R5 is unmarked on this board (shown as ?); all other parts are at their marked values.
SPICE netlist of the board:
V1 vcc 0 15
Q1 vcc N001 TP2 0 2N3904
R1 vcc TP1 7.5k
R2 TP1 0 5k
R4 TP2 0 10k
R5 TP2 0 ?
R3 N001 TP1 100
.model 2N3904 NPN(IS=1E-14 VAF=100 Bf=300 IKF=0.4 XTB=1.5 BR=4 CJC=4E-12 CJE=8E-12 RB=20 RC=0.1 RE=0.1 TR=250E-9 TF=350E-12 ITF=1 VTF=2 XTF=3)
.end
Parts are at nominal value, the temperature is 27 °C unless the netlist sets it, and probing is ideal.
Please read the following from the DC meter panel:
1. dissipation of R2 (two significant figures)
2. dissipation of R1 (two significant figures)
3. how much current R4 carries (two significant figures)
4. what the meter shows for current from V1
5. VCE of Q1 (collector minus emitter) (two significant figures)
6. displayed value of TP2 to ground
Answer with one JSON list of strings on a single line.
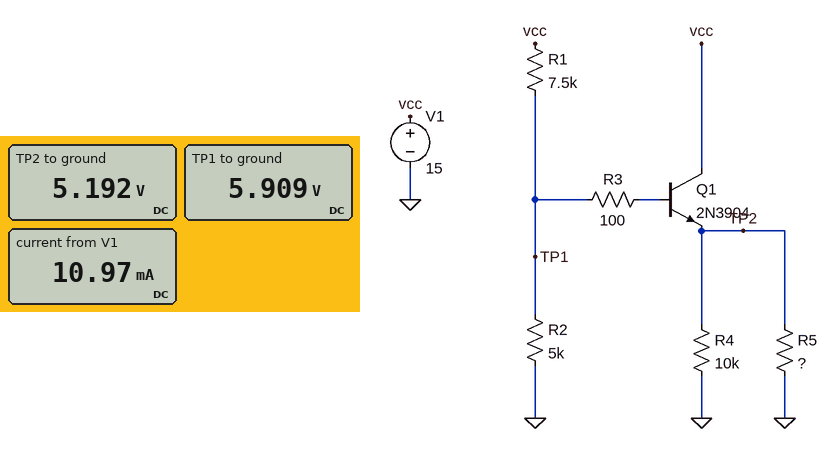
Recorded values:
["7.0 mW", "11 mW", "520 µA", "10.97 mA", "9.8 V", "5.192 V"]
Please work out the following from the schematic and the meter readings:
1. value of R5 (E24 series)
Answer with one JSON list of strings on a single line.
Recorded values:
["560 Ω"]
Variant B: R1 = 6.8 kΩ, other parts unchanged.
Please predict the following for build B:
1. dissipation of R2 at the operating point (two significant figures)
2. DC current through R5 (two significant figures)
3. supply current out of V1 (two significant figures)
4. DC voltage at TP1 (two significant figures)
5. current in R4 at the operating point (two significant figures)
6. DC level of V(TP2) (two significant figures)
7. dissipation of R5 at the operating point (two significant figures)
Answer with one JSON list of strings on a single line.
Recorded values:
["7.8 mW", "9.9 mA", "12 mA", "6.3 V", "550 µA", "5.5 V", "55 mW"]
